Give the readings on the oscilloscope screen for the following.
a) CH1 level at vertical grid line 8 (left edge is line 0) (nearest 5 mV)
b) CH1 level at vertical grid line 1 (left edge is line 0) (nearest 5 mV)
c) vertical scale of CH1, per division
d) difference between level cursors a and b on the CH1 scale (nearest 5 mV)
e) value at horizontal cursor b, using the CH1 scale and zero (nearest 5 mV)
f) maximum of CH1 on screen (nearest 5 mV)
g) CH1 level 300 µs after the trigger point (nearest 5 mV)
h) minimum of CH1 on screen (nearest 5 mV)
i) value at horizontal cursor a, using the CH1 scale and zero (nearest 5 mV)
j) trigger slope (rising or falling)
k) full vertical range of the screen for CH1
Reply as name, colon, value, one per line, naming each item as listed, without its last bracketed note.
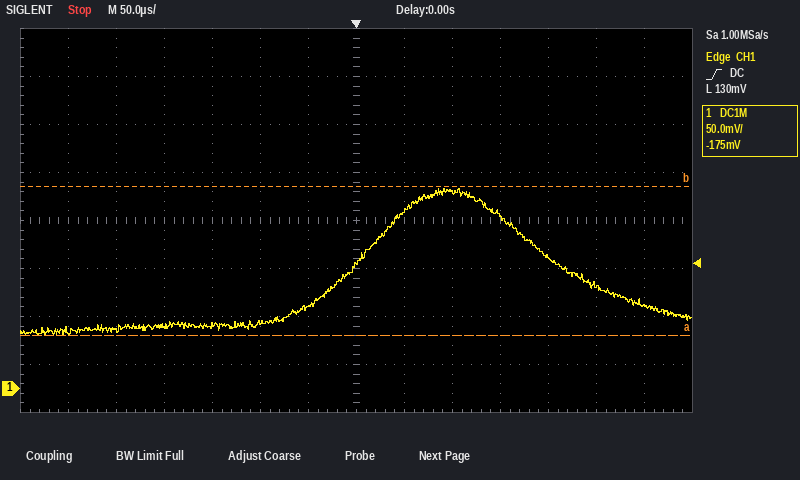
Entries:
CH1 level at vertical grid line 8 (left edge is line 0): 185 mV
CH1 level at vertical grid line 1 (left edge is line 0): 60 mV
vertical scale of CH1, per division: 50 mV
difference between level cursors a and b on the CH1 scale: 155 mV
value at horizontal cursor b, using the CH1 scale and zero: 210 mV
maximum of CH1 on screen: 210 mV
CH1 level 300 µs after the trigger point: 85 mV
minimum of CH1 on screen: 55 mV
value at horizontal cursor a, using the CH1 scale and zero: 55 mV
trigger slope: rising
full vertical range of the screen for CH1: 400 mV
